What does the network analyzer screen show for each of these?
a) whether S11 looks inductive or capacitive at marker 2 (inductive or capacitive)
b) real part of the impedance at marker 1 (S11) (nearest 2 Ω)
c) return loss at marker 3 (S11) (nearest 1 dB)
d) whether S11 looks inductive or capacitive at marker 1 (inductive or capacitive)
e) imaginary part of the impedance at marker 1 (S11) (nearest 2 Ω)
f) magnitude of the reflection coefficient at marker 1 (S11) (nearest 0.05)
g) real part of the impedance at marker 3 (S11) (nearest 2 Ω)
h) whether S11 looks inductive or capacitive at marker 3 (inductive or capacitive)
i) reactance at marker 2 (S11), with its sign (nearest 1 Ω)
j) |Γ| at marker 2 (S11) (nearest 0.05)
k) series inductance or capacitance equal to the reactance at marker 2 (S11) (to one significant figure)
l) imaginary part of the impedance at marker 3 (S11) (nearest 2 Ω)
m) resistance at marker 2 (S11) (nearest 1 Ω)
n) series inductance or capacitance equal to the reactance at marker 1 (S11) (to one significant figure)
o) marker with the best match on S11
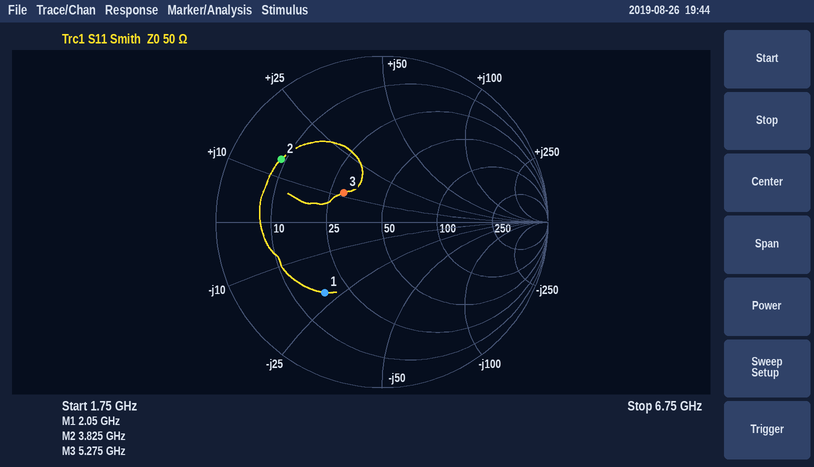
inductive
18 Ω
11 dB
capacitive
-22 Ω
0.55
30 Ω
inductive
+14 Ω
0.70
600 pH
+12 Ω
9 Ω
4 pF
marker 3
